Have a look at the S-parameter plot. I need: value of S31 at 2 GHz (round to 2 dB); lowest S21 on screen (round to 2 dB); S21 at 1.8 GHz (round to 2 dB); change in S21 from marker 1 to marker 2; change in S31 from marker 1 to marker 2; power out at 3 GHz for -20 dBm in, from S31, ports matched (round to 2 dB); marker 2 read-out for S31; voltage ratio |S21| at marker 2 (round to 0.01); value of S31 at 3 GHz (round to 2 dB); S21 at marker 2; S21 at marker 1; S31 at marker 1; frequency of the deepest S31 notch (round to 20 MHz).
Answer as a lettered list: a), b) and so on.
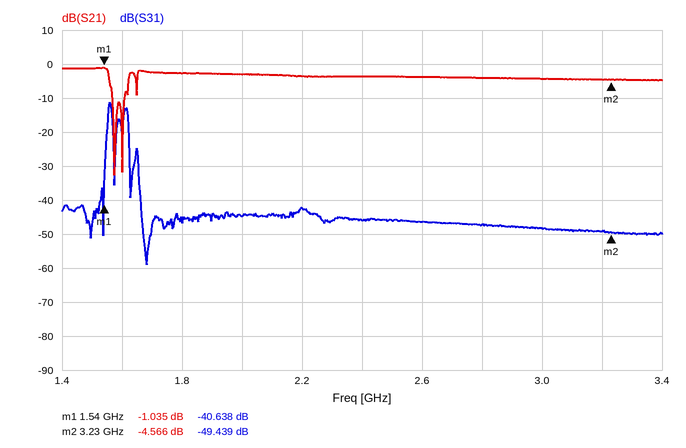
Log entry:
a) -44 dB
b) -32 dB
c) -2 dB
d) -3.531 dB
e) -8.801 dB
f) -68 dBm
g) -49.439 dB
h) 0.59
i) -48 dB
j) -4.566 dB
k) -1.035 dB
l) -40.638 dB
m) 1.68 GHz
